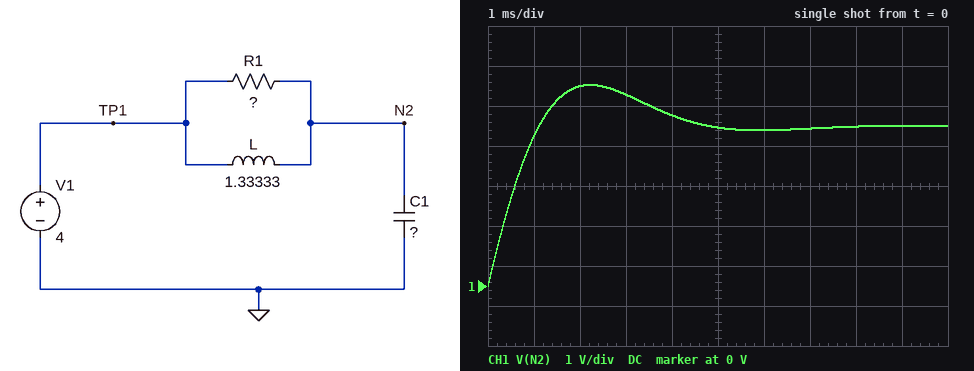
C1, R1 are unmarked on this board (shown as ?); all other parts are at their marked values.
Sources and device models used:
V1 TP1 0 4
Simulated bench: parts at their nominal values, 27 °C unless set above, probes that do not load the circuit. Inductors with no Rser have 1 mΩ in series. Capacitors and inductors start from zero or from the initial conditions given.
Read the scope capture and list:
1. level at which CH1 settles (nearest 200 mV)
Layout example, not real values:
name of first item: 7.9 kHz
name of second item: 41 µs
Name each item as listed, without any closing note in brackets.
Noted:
level at which CH1 settles: 4.0 V
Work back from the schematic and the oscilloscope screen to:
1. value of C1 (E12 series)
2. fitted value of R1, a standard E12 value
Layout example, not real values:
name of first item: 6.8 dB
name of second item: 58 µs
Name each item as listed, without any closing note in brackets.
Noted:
value of C1: 680 nF
fitted value of R1, a standard E12 value: 1.2 kΩ
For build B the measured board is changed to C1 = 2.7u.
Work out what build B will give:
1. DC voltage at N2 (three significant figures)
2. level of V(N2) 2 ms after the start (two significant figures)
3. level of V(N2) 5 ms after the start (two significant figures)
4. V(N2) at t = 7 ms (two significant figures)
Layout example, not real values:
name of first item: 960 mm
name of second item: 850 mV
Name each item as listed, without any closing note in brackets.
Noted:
DC voltage at N2: 4.00 V
level of V(N2) 2 ms after the start: 3.2 V
level of V(N2) 5 ms after the start: 5.8 V
V(N2) at t = 7 ms: 5.1 V
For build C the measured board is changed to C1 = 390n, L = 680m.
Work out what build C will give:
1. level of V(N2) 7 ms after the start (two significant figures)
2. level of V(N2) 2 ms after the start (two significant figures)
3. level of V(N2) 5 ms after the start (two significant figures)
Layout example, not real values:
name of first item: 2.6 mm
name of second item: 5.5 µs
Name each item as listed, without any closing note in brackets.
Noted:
level of V(N2) 7 ms after the start: 4.0 V
level of V(N2) 2 ms after the start: 4.4 V
level of V(N2) 5 ms after the start: 4.0 V
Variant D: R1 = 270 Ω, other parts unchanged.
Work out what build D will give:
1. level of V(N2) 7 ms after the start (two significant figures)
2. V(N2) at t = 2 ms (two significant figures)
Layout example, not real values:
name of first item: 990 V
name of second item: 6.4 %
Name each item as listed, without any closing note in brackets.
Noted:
level of V(N2) 7 ms after the start: 4.0 V
V(N2) at t = 2 ms: 4.1 V
